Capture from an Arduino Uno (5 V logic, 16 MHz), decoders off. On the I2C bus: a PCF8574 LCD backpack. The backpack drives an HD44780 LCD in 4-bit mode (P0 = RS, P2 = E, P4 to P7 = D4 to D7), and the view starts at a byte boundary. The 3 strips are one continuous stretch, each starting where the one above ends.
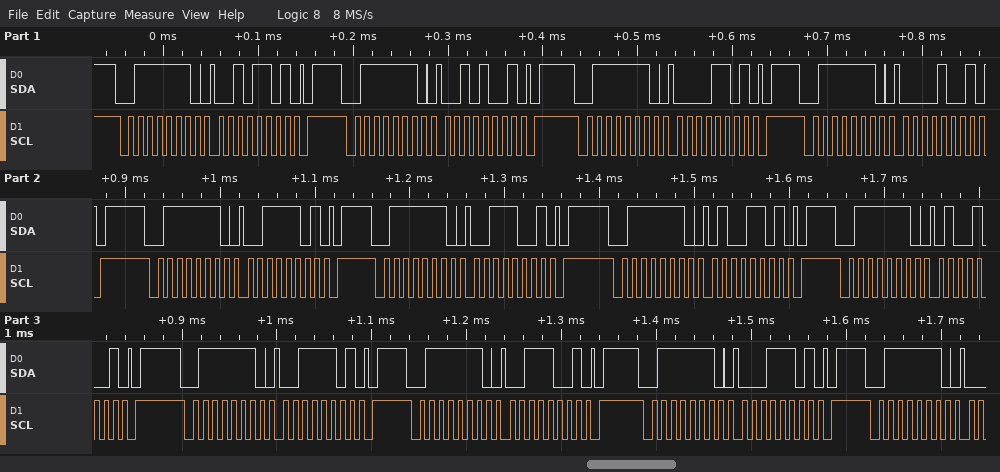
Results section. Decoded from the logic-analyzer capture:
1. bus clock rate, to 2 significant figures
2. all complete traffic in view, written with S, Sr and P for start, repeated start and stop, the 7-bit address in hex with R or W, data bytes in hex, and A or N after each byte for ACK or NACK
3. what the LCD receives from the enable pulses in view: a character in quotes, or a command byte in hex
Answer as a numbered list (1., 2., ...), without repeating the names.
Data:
1. 100 kHz
2. S 3FW A 2D A P S 3FW A 29 A P S 3FW A 0D A P S 3FW A 09 A P S 3FW A 3D A P S 3FW A 39 A P S 3FW A 4D A P S 3FW A 49 A P S 3FW A 3D A P S 3FW A 39 A P S 3FW A 1D A P S 3FW A
3. ' ' '4'
